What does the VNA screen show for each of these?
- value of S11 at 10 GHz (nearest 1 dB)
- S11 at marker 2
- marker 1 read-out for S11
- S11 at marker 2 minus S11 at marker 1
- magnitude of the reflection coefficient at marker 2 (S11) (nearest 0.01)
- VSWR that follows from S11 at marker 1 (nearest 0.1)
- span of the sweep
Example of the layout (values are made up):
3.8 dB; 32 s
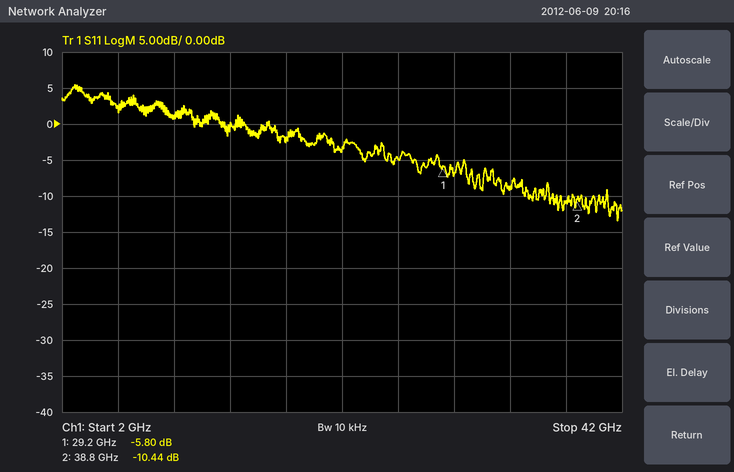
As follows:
1 dB; -10.44 dB; -5.80 dB; -4.64 dB; 0.30; 3.1; 40 GHz
